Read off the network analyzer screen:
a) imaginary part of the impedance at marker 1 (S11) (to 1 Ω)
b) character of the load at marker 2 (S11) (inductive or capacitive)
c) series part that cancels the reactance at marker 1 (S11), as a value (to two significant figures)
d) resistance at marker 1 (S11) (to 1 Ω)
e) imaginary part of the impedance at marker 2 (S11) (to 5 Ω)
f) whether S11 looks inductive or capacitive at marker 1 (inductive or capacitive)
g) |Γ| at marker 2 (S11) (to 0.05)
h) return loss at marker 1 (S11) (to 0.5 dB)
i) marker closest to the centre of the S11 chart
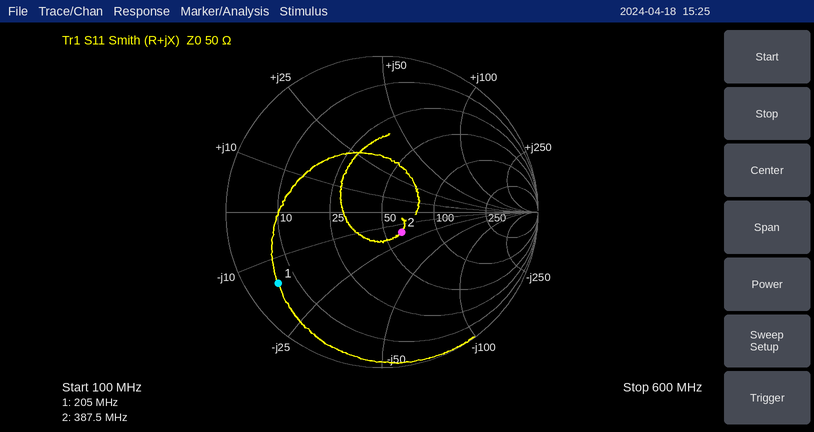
-15 Ω
capacitive
12 nH
6 Ω
-15 Ω
capacitive
0.20
2.0 dB
marker 2
